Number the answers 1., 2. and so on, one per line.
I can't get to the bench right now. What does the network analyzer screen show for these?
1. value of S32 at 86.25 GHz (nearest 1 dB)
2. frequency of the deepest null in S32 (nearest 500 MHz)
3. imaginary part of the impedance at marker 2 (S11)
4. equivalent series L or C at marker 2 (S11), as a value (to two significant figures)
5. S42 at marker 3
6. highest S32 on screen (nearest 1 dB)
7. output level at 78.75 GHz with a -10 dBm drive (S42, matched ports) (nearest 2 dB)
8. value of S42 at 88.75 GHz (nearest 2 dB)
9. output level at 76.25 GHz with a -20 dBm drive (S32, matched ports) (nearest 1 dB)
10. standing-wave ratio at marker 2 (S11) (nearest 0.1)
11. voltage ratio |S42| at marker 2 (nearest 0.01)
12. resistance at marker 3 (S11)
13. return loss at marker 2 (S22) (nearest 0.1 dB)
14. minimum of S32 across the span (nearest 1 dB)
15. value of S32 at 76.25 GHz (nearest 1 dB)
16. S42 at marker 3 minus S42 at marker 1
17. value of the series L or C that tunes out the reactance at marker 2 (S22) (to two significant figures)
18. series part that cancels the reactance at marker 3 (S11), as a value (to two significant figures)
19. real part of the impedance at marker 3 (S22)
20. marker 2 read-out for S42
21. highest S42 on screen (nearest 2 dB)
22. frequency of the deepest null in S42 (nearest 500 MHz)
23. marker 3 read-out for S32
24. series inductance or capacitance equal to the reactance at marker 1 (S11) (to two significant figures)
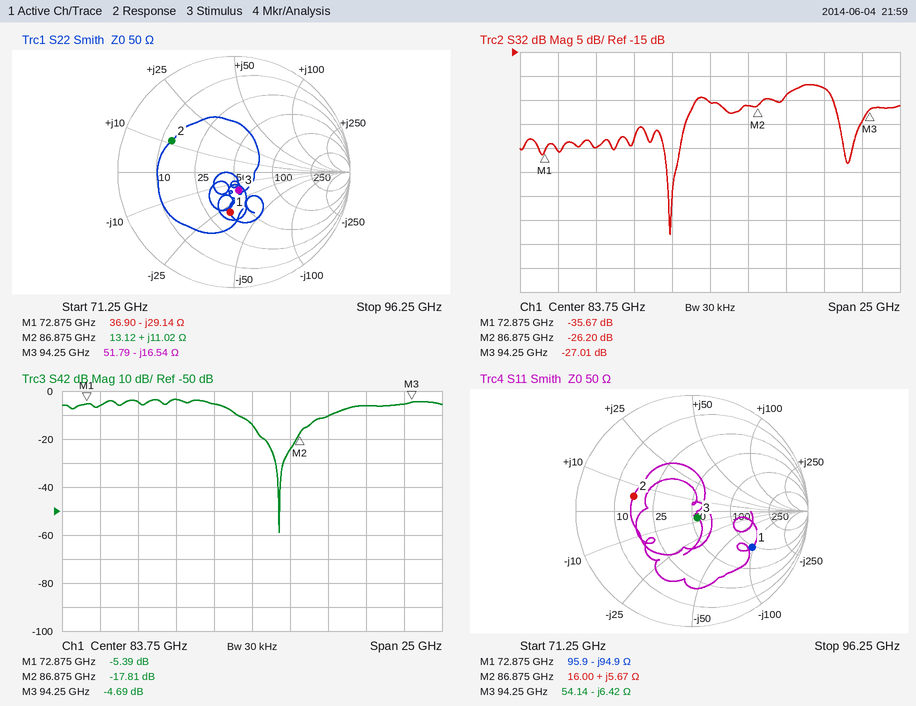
1. -26 dB
2. 81.0 GHz
3. +5.67 Ω
4. 10 pH
5. -4.69 dB
6. -22 dB
7. -14 dBm
8. -10 dB
9. -55 dBm
10. 3.2
11. 0.13
12. 54.14 Ω
13. 4.4 dB
14. -53 dB
15. -35 dB
16. 0.70 dB
17. 170 fF
18. 11 pH
19. 51.79 Ω
20. -17.81 dB
21. -4 dB
22. 85.5 GHz
23. -27.01 dB
24. 23 fF
